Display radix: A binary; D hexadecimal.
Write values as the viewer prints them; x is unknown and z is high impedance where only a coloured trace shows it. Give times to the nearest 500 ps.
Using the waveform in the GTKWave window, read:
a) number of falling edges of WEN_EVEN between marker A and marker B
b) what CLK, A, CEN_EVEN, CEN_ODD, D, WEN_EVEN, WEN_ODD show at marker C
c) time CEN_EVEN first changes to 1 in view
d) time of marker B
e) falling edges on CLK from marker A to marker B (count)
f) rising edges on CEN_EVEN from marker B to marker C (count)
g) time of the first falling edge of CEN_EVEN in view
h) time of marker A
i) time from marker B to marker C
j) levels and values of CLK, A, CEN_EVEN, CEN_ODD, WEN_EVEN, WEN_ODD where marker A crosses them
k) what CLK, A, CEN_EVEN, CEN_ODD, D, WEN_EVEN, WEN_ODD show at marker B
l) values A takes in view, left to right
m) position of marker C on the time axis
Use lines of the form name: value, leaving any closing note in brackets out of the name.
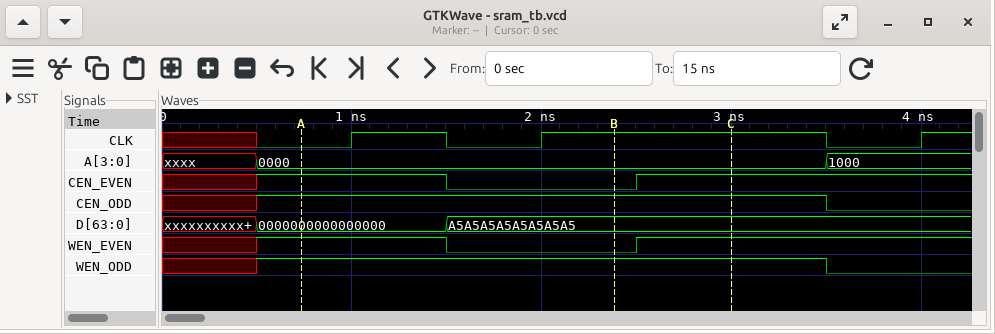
number of falling edges of WEN_EVEN between marker A and marker B: 1
what CLK, A, CEN_EVEN, CEN_ODD, D, WEN_EVEN, WEN_ODD show at marker C: CLK=1, A=0000, CEN_EVEN=1, CEN_ODD=1, D=A5A5A5A5A5A5A5A5, WEN_EVEN=1, WEN_ODD=1
time CEN_EVEN first changes to 1 in view: 500 ps
time of marker B: 2500 ps
falling edges on CLK from marker A to marker B: 1
rising edges on CEN_EVEN from marker B to marker C: 1
time of the first falling edge of CEN_EVEN in view: 1500 ps
time of marker A: 500 ps
time from marker B to marker C: 500 ps
levels and values of CLK, A, CEN_EVEN, CEN_ODD, WEN_EVEN, WEN_ODD where marker A crosses them: CLK=0, A=0000, CEN_EVEN=1, CEN_ODD=1, WEN_EVEN=1, WEN_ODD=1
what CLK, A, CEN_EVEN, CEN_ODD, D, WEN_EVEN, WEN_ODD show at marker B: CLK=1, A=0000, CEN_EVEN=0, CEN_ODD=1, D=A5A5A5A5A5A5A5A5, WEN_EVEN=0, WEN_ODD=1
values A takes in view, left to right: xxxx, 0000, 1000
position of marker C on the time axis: 3000 ps
